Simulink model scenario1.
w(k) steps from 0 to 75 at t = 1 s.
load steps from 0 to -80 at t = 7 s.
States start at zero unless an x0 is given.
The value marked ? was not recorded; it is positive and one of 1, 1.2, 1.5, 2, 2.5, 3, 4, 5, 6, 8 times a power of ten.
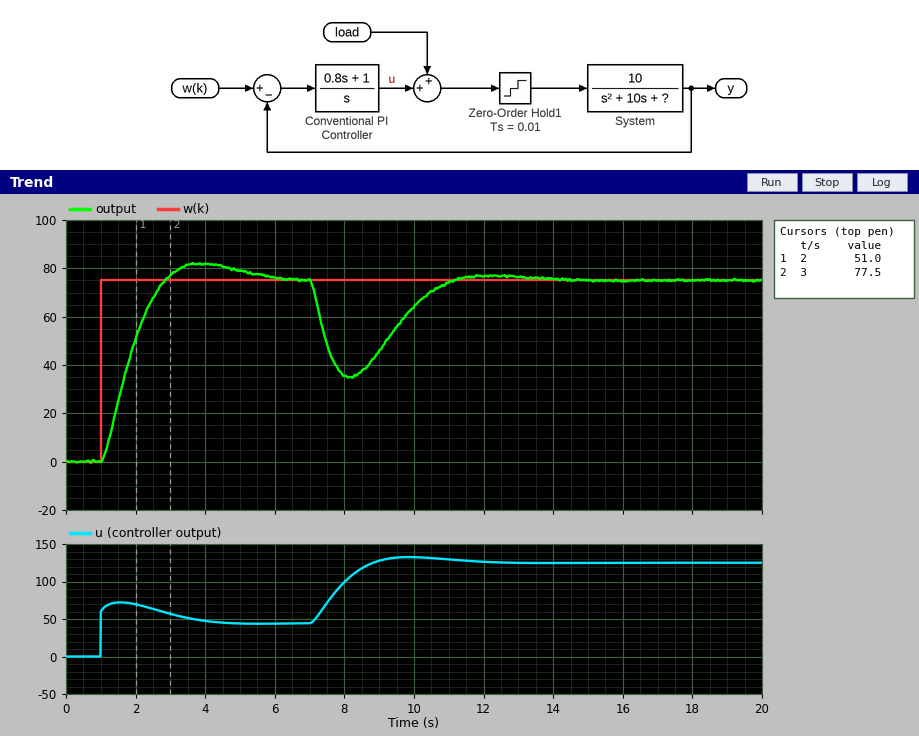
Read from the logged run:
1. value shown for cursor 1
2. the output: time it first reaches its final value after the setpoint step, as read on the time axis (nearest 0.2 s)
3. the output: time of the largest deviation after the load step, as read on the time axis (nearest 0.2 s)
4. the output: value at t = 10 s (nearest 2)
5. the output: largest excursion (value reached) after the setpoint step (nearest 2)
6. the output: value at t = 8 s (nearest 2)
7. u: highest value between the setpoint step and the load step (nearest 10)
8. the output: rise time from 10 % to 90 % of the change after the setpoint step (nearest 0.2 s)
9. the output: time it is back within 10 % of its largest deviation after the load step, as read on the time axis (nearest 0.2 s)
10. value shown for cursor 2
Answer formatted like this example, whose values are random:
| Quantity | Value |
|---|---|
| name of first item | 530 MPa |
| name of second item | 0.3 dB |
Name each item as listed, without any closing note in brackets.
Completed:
| Quantity | Value |
|---|---|
| value shown for cursor 1 | 51.0 |
| the output: time it first reaches its final value after the setpoint step, as read on the time axis | 2.8 s |
| the output: time of the largest deviation after the load step, as read on the time axis | 8.2 s |
| the output: value at t = 10 s | 64 |
| the output: largest excursion (value reached) after the setpoint step | 82 |
| the output: value at t = 8 s | 36 |
| u: highest value between the setpoint step and the load step | 70 |
| the output: rise time from 10 % to 90 % of the change after the setpoint step | 1.2 s |
| the output: time it is back within 10 % of its largest deviation after the load step, as read on the time axis | 10.6 s |
| value shown for cursor 2 | 77.5 |
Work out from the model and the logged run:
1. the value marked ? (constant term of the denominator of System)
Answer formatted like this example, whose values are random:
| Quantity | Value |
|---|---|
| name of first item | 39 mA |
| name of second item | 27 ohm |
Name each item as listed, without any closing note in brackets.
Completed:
| Quantity | Value |
|---|---|
| the value marked ? | 6 |
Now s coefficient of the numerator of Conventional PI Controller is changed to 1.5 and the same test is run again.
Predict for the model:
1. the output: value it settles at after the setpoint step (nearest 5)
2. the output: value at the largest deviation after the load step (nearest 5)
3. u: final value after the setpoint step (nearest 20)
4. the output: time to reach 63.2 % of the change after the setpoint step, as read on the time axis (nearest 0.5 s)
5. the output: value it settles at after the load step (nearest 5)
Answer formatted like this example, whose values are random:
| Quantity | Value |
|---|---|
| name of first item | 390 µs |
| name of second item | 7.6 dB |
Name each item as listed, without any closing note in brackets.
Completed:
| Quantity | Value |
|---|---|
| the output: value it settles at after the setpoint step | 75 |
| the output: value at the largest deviation after the load step | 45 |
| u: final value after the setpoint step | 40 |
| the output: time to reach 63.2 % of the change after the setpoint step, as read on the time axis | 1.5 s |
| the output: value it settles at after the load step | 75 |
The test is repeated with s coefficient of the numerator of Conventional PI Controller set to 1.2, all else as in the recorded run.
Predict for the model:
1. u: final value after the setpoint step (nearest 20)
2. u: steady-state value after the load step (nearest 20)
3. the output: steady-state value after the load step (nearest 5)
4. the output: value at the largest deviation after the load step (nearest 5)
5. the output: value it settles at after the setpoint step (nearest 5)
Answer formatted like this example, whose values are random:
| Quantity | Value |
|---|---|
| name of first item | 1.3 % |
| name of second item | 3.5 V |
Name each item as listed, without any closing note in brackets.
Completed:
| Quantity | Value |
|---|---|
| u: final value after the setpoint step | 40 |
| u: steady-state value after the load step | 120 |
| the output: steady-state value after the load step | 75 |
| the output: value at the largest deviation after the load step | 40 |
| the output: value it settles at after the setpoint step | 75 |
